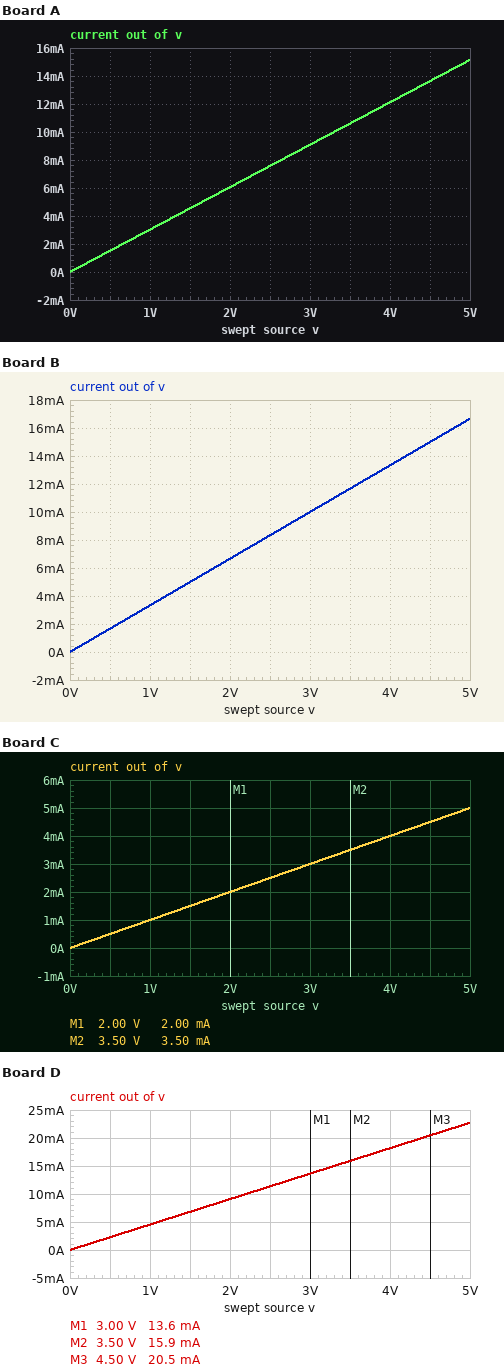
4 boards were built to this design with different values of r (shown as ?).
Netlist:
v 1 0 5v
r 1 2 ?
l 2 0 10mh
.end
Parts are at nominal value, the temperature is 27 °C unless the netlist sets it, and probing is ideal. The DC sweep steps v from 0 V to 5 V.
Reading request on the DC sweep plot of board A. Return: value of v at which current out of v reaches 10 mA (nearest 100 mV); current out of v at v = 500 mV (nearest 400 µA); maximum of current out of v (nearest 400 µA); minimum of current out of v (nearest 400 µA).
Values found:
3.3 V
1.6 mA
15.2 mA
0 A
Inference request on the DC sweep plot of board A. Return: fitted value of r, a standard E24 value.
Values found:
330 Ω
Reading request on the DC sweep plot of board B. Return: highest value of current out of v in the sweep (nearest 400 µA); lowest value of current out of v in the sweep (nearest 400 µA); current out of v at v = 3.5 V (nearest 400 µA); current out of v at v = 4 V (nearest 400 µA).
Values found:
16.8 mA
0 A
11.6 mA
13.2 mA
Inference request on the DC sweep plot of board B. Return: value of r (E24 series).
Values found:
300 Ω
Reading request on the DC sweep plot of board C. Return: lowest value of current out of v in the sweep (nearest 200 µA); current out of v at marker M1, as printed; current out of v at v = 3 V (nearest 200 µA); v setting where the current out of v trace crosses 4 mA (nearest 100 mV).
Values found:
0 A
2.00 mA
3.0 mA
4.0 V
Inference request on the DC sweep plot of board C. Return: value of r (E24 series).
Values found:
1 kΩ
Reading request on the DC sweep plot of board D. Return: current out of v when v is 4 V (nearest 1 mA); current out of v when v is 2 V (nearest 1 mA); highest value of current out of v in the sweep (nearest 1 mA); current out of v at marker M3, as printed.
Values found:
18 mA
9 mA
23 mA
20.5 mA
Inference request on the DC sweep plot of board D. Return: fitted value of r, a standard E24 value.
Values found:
220 Ω
